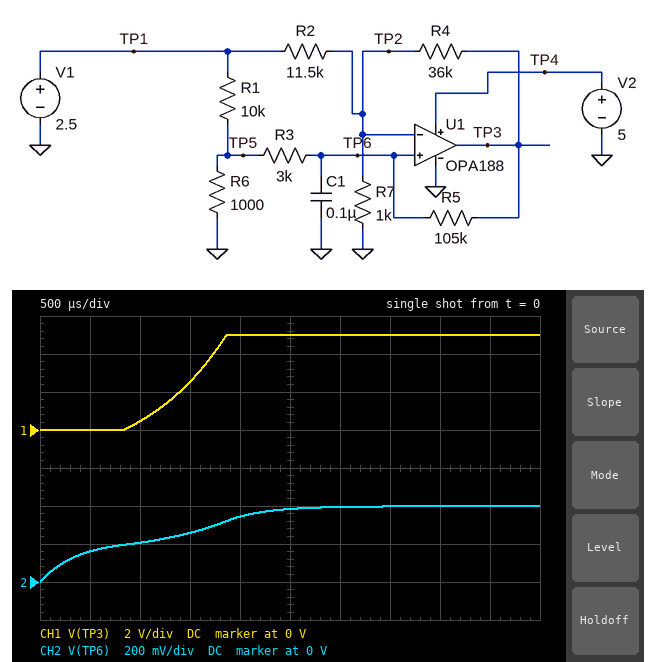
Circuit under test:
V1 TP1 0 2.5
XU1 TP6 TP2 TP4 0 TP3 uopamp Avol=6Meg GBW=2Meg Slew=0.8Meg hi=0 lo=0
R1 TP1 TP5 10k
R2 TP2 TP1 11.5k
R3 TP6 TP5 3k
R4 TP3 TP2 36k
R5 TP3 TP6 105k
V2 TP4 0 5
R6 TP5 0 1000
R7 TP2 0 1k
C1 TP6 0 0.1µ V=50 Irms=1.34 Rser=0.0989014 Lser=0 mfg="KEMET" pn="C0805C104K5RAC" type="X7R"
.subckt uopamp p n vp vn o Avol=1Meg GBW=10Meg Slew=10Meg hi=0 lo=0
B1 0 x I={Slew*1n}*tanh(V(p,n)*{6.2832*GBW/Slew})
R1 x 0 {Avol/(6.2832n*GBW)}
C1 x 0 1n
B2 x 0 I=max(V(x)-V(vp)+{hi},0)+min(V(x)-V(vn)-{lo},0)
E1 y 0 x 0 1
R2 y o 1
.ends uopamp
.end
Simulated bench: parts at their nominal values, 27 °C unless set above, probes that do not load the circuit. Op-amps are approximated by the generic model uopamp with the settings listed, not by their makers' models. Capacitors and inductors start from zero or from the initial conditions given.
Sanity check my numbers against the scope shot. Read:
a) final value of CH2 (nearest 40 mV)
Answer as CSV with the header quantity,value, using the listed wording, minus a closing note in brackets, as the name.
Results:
quantity,value
final value of CH2,400 mV
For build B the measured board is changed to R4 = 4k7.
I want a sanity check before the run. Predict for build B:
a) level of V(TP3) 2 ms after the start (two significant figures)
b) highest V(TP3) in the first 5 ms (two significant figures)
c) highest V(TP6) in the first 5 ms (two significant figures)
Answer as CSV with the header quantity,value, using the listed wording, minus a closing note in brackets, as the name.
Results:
quantity,value
level of V(TP3) 2 ms after the start,390 mV
highest V(TP3) in the first 5 ms,410 mV
highest V(TP6) in the first 5 ms,230 mV
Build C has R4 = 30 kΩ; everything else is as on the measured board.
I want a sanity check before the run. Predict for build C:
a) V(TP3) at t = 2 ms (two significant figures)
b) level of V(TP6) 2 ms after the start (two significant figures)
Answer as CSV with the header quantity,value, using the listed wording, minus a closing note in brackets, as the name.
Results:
quantity,value
V(TP3) at t = 2 ms,3.7 V
level of V(TP6) 2 ms after the start,300 mV
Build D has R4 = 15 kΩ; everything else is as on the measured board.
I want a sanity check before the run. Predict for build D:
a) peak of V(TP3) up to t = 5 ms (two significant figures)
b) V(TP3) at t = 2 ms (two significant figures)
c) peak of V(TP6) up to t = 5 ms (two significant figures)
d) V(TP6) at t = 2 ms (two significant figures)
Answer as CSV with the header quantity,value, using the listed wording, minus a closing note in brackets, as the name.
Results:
quantity,value
peak of V(TP3) up to t = 5 ms,1.4 V
V(TP3) at t = 2 ms,1.0 V
peak of V(TP6) up to t = 5 ms,270 mV
V(TP6) at t = 2 ms,250 mV
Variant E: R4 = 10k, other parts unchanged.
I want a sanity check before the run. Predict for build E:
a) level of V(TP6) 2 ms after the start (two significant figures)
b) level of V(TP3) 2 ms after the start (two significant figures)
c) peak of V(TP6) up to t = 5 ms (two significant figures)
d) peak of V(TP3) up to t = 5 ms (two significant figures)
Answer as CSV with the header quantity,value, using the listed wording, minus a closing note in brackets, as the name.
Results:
quantity,value
level of V(TP6) 2 ms after the start,240 mV
level of V(TP3) 2 ms after the start,640 mV
peak of V(TP6) up to t = 5 ms,250 mV
peak of V(TP3) up to t = 5 ms,740 mV
